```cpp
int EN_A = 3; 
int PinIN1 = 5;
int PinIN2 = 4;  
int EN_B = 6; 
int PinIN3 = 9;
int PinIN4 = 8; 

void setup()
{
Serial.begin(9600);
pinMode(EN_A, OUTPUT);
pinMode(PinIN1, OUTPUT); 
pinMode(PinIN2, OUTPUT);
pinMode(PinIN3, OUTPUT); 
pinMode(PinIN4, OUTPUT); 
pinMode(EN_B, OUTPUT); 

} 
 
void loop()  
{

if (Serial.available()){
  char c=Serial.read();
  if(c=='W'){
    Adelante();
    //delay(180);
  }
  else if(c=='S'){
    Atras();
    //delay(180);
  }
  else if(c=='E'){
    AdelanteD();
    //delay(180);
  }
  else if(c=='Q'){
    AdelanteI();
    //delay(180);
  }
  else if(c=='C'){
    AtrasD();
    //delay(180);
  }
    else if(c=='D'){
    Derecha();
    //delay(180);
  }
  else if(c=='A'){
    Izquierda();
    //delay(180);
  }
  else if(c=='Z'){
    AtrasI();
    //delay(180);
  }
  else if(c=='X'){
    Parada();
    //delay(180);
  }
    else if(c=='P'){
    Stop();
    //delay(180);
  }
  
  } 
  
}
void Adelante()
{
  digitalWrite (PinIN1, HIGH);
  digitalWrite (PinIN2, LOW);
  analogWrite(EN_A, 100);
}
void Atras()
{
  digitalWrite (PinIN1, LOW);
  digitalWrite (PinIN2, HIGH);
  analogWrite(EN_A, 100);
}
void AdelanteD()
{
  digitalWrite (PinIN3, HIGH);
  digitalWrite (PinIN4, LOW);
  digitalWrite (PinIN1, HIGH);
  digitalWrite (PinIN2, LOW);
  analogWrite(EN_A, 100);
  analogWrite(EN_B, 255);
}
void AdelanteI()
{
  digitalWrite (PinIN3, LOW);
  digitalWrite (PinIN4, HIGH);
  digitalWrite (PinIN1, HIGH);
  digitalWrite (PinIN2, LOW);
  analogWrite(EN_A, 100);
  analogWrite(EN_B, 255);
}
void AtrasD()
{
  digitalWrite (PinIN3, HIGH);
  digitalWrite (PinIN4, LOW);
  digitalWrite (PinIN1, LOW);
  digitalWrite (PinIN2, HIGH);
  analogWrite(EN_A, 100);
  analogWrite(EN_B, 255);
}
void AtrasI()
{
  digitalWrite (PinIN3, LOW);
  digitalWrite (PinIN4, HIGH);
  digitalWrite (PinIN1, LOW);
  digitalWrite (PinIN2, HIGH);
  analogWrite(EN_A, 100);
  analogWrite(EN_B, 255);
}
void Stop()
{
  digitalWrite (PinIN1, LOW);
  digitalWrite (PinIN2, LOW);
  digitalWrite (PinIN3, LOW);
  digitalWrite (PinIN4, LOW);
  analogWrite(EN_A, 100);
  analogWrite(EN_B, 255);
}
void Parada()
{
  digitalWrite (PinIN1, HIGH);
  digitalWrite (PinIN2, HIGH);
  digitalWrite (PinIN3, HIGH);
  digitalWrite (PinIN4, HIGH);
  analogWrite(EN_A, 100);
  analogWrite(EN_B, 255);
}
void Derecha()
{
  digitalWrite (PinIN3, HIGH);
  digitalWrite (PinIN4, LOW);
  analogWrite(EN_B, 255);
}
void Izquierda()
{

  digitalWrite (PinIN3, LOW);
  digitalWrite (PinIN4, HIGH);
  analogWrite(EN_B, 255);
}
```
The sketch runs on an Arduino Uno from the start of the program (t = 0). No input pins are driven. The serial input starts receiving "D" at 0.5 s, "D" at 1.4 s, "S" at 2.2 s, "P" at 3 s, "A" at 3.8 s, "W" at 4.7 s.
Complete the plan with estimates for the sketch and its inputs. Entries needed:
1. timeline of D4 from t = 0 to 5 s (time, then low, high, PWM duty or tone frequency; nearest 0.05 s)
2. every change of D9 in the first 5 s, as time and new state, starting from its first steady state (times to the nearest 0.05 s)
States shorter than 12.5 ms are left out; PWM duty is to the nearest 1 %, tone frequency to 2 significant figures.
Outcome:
0 s low; 2.2 s high; 3 s low
0 s low; 0.5 s high; 3 s low
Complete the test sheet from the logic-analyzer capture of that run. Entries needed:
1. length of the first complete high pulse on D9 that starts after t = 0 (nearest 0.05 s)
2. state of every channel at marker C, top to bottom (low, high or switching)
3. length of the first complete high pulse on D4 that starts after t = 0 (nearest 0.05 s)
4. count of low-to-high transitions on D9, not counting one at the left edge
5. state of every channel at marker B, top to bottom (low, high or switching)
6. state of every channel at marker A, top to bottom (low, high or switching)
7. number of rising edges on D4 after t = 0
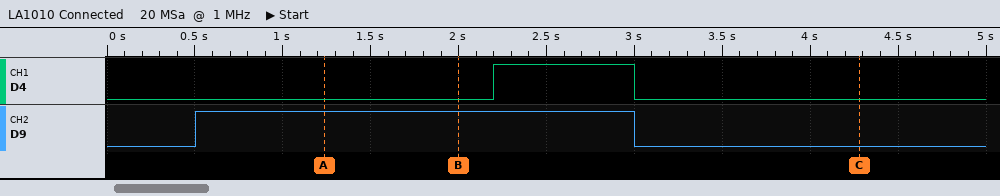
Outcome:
2.50 s
D4 low, D9 low
0.80 s
1
D4 low, D9 high
D4 low, D9 high
1
